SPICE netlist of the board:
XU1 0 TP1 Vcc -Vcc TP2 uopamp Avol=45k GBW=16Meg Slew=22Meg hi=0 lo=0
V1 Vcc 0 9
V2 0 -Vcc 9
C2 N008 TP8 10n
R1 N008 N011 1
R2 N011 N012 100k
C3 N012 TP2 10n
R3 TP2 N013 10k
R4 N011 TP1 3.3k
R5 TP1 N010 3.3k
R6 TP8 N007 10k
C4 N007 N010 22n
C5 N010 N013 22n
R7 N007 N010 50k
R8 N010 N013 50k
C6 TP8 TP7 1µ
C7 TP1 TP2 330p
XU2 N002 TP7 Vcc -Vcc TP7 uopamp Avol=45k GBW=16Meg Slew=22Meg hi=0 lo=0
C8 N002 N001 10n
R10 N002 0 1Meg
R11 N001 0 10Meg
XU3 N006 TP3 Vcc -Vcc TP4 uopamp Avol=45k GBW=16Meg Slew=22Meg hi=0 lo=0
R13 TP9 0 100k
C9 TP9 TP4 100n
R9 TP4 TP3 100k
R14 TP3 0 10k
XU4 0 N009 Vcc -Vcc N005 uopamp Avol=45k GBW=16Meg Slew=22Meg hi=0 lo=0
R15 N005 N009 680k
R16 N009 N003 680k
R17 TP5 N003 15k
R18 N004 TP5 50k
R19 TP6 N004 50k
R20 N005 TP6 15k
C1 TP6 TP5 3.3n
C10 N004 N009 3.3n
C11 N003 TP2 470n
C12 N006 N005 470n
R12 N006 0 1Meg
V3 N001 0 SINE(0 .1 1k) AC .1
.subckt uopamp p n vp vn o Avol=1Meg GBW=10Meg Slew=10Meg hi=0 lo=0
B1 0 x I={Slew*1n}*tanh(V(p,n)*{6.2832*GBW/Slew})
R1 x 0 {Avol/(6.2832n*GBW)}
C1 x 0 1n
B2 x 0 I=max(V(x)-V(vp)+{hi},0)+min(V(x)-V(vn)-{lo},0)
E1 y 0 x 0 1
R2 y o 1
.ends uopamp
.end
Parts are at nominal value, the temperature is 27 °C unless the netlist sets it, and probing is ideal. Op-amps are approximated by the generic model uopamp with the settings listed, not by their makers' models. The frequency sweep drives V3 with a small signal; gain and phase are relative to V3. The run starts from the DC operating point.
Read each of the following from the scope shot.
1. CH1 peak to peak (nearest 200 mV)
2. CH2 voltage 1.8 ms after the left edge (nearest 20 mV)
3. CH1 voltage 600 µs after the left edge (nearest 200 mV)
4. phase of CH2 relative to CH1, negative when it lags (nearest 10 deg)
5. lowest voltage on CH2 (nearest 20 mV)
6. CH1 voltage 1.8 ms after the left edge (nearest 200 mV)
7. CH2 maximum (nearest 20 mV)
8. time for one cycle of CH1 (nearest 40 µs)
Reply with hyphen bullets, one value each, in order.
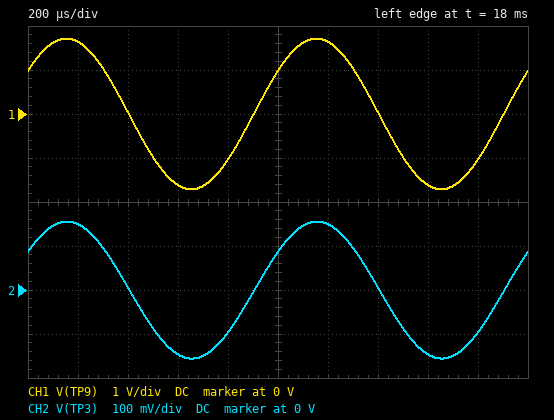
- 3.4 V
- -100 mV
- -1.6 V
- 0 deg
- -160 mV
- -1.0 V
- 160 mV
- 1.00 ms
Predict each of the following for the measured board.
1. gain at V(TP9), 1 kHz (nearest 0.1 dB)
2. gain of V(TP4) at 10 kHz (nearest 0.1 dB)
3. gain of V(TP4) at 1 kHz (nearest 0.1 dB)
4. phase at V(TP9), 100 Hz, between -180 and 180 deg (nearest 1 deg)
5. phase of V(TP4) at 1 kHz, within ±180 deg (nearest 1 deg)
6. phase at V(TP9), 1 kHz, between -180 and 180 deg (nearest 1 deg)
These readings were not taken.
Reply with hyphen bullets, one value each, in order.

- 24.7 dB
- 34.8 dB
- 24.7 dB
- 31 deg
- 34 deg
- 35 deg
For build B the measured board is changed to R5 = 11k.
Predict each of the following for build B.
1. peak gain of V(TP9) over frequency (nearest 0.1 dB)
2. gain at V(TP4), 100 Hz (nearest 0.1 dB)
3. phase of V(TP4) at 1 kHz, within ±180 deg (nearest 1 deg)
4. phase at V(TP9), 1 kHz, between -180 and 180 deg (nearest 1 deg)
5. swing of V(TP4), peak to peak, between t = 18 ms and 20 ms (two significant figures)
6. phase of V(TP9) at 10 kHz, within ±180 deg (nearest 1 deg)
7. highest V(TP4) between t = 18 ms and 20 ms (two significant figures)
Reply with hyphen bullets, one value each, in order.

- 38.8 dB
- 19.8 dB
- 48 deg
- 49 deg
- 4.2 V
- -4 deg
- 2.1 V
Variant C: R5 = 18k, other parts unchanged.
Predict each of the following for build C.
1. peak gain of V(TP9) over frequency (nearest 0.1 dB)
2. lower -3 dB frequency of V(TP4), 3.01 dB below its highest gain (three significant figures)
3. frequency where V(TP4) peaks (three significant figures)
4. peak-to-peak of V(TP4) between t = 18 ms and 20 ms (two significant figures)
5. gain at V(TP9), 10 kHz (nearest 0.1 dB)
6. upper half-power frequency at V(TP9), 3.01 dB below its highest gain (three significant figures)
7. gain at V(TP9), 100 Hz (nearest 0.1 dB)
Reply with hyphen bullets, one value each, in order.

- 40.8 dB
- 3.94 kHz
- 8.78 kHz
- 4.9 V
- 40.7 dB
- 19.5 kHz
- 19.6 dB
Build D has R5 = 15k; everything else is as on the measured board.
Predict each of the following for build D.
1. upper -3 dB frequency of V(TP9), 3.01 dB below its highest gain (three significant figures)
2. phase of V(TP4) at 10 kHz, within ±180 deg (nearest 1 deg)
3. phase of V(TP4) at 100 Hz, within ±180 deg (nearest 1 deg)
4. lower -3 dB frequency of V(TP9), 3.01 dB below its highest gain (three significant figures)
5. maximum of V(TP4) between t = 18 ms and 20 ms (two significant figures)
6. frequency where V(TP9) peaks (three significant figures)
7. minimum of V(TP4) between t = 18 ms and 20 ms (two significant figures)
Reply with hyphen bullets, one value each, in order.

- 21.1 kHz
- -8 deg
- 24 deg
- 3.99 kHz
- 2.3 V
- 9.20 kHz
- -2.3 V
